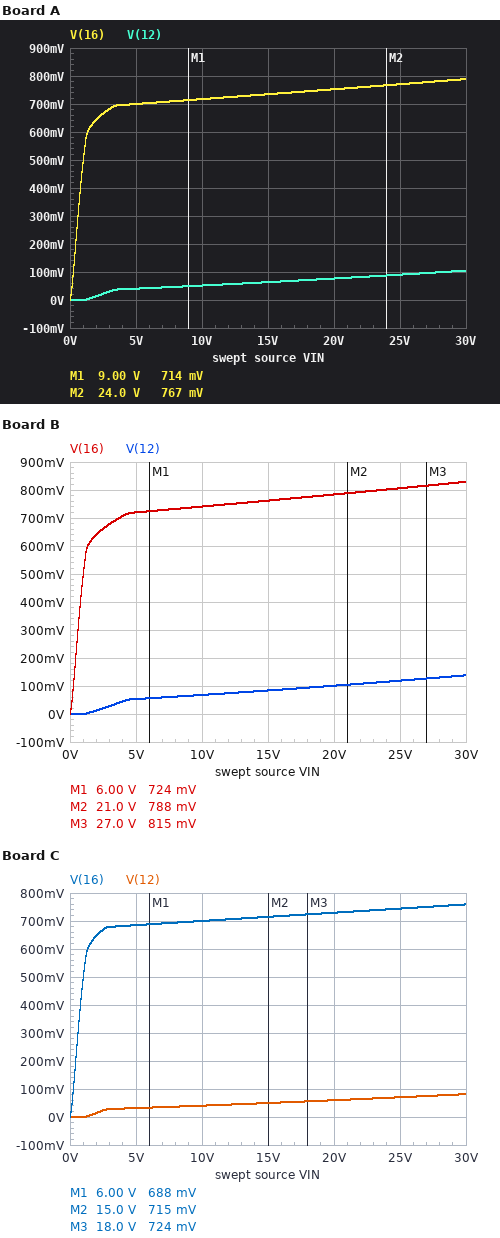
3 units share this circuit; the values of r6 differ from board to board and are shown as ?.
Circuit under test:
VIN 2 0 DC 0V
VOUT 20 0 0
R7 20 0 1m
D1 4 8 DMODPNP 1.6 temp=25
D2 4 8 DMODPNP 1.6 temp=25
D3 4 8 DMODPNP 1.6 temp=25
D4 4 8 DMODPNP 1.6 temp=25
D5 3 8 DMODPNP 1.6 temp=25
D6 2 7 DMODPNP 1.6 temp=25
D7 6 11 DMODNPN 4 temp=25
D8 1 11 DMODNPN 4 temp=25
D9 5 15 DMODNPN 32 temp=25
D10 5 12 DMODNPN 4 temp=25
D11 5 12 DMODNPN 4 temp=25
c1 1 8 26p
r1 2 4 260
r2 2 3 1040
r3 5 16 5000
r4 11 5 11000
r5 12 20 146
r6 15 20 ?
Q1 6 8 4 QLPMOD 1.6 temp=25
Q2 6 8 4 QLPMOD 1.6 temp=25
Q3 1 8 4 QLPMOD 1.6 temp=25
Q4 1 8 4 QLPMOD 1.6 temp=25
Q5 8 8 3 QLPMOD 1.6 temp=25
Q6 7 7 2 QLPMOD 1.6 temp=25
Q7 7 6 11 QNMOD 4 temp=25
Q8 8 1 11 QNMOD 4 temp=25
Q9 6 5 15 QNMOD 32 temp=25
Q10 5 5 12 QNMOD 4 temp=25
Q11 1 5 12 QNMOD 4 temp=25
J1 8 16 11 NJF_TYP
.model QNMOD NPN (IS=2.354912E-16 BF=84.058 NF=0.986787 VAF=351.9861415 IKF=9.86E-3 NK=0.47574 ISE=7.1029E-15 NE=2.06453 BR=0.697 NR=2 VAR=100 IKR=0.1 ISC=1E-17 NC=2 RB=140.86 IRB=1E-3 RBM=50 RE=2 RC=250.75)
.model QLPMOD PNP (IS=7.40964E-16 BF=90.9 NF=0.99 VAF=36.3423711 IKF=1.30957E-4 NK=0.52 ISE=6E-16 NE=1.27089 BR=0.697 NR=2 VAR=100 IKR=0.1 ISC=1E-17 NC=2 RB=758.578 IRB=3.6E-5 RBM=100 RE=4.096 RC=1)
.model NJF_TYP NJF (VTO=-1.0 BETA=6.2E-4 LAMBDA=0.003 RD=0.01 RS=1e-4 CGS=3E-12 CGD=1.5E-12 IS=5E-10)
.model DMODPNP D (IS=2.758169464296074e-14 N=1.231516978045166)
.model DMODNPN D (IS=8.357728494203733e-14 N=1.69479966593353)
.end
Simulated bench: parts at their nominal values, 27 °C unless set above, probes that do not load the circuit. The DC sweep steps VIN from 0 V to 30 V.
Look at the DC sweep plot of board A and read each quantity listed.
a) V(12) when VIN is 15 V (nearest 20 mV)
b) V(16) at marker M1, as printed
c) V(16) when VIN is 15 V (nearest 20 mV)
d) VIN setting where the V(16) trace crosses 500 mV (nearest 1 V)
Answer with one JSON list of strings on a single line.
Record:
["60 mV", "714 mV", "740 mV", "1 V"]
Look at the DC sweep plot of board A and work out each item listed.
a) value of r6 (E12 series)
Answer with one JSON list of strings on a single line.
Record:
["330 Ω"]
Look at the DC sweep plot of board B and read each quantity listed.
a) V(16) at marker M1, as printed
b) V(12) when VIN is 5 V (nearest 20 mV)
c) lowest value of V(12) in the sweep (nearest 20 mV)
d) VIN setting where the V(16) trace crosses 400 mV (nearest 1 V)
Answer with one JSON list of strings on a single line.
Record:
["724 mV", "60 mV", "0 V", "1 V"]
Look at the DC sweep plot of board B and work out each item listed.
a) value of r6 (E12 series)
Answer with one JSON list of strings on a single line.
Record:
["270 Ω"]
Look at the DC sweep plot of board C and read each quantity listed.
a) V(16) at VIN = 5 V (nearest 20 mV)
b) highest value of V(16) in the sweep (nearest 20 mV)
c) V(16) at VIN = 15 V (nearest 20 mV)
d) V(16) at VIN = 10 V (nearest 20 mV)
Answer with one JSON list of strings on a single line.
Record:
["680 mV", "760 mV", "720 mV", "700 mV"]
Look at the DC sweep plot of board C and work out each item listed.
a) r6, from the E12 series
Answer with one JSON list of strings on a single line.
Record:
["390 Ω"]
